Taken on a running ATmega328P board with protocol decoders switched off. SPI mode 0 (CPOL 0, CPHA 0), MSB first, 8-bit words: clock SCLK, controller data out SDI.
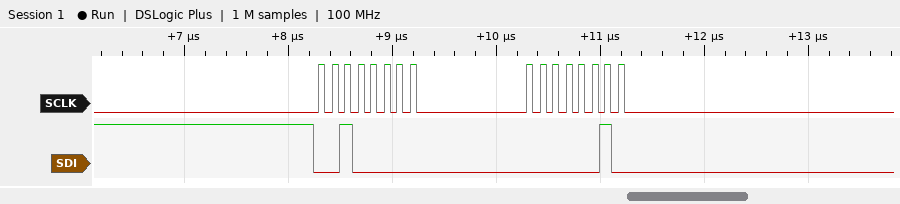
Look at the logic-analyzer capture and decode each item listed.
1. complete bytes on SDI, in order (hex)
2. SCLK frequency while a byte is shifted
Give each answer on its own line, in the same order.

0x20 0x02
8 MHz
